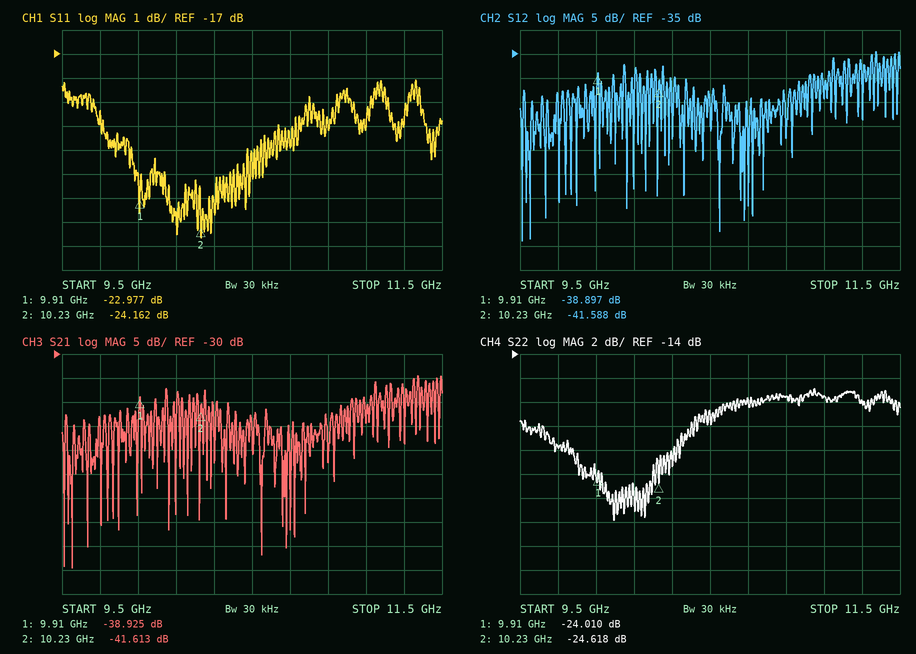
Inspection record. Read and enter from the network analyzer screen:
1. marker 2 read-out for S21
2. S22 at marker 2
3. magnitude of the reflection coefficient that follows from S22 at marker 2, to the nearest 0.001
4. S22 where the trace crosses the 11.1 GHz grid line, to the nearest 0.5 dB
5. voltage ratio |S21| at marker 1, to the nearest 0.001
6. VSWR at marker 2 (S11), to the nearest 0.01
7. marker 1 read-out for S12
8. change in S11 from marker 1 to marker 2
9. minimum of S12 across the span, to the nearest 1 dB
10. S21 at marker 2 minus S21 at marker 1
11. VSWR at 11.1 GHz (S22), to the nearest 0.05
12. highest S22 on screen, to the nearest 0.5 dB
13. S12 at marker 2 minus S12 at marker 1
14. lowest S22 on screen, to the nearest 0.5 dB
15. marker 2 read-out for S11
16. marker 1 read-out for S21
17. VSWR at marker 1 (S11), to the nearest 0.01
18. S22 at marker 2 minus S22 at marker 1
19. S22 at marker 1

-41.613 dB
-24.618 dB
0.059
-17.5 dB
0.011
1.13
-38.897 dB
-1.185 dB
-74 dB
-2.688 dB
1.30
-17.0 dB
-2.691 dB
-28.0 dB
-24.162 dB
-38.925 dB
1.15
-0.608 dB
-24.010 dB
